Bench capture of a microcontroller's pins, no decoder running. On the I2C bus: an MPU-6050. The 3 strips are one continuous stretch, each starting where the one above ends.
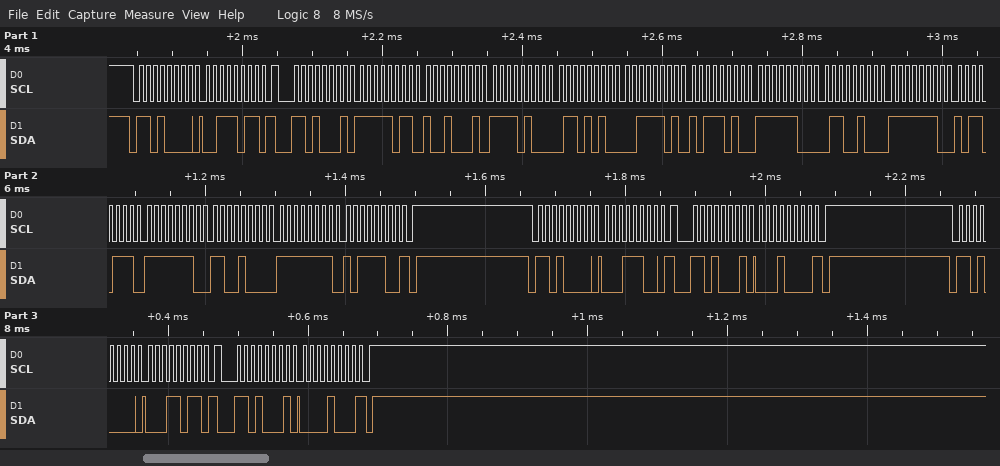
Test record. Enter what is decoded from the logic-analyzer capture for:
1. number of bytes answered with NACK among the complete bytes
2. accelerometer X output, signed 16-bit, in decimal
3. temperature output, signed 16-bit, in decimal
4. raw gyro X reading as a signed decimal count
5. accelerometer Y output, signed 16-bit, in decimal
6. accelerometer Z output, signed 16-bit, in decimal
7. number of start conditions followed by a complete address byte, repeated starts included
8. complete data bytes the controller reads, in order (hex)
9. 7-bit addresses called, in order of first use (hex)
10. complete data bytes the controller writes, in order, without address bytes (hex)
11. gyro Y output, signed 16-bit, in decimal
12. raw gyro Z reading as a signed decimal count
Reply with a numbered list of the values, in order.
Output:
1. 3
2. -1135
3. -924
4. -329
5. -2966
6. 15802
7. 6
8. FB 91 F4 6A 3D BA FC 64 FE B7 FE C8 FF BC 10 08
9. 0x68
10. 3B 1C 1B
11. -312
12. -68
